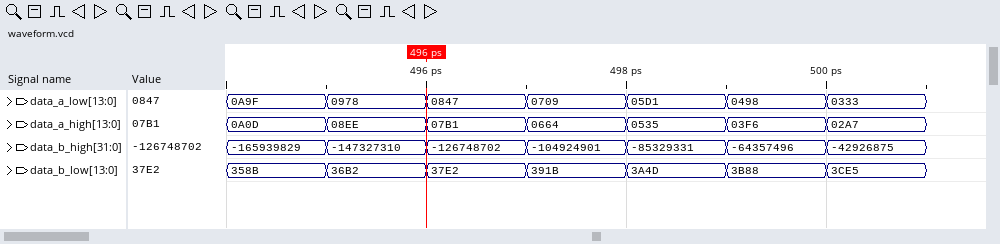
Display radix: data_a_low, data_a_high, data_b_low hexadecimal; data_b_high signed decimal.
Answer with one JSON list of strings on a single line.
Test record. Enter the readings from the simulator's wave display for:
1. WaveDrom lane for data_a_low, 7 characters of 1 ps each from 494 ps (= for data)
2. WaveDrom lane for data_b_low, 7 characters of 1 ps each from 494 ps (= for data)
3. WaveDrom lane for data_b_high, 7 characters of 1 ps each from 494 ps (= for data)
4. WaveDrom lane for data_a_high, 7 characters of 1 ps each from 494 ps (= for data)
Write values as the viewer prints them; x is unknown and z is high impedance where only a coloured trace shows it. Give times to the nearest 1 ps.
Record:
["{name: 'data_a_low', wave: '=======', data: '0A9F 0978 0847 0709 05D1 0498 0333'}", "{name: 'data_b_low', wave: '=======', data: '358B 36B2 37E2 391B 3A4D 3B88 3CE5'}", "{name: 'data_b_high', wave: '=======', data: '-165939829 -147327310 -126748702 -104924901 -85329331 -64357496 -42926875'}", "{name: 'data_a_high', wave: '=======', data: '0A0D 08EE 07B1 0664 0535 03F6 02A7'}"]
